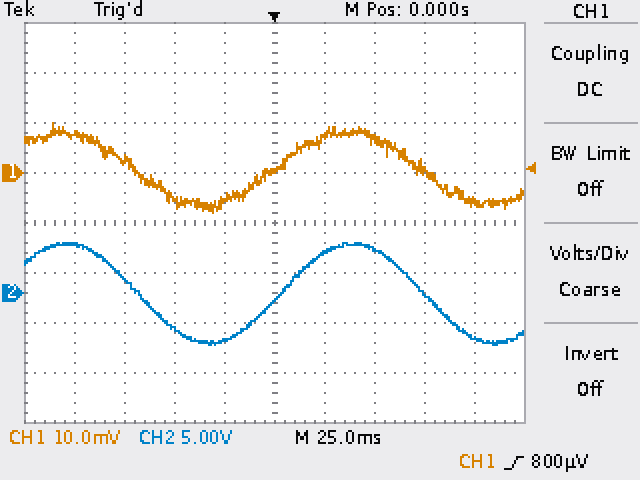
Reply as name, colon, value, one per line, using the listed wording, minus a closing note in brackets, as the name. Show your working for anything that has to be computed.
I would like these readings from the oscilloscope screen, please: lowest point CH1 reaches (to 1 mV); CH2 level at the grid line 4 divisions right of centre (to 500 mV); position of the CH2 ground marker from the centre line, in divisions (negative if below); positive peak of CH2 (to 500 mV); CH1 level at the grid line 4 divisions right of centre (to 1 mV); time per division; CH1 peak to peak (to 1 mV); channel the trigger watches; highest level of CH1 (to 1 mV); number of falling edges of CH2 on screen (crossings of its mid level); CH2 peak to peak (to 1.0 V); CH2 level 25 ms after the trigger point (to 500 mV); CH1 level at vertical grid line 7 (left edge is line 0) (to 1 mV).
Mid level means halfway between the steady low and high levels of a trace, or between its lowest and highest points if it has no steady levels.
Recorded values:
lowest point CH1 reaches: -8 mV
CH2 level at the grid line 4 divisions right of centre: -4.5 V
position of the CH2 ground marker from the centre line, in divisions: -1.4 div
positive peak of CH2: 5.0 V
CH1 level at the grid line 4 divisions right of centre: -6 mV
time per division: 25 ms
CH1 peak to peak: 10 mV − (-8 mV) = 18 mV
channel the trigger watches: CH1
highest level of CH1: 10 mV
number of falling edges of CH2 on screen: 2
CH2 peak to peak: 10.0 V
CH2 level 25 ms after the trigger point: 4.0 V
CH1 level at vertical grid line 7 (left edge is line 0): 7 mV
